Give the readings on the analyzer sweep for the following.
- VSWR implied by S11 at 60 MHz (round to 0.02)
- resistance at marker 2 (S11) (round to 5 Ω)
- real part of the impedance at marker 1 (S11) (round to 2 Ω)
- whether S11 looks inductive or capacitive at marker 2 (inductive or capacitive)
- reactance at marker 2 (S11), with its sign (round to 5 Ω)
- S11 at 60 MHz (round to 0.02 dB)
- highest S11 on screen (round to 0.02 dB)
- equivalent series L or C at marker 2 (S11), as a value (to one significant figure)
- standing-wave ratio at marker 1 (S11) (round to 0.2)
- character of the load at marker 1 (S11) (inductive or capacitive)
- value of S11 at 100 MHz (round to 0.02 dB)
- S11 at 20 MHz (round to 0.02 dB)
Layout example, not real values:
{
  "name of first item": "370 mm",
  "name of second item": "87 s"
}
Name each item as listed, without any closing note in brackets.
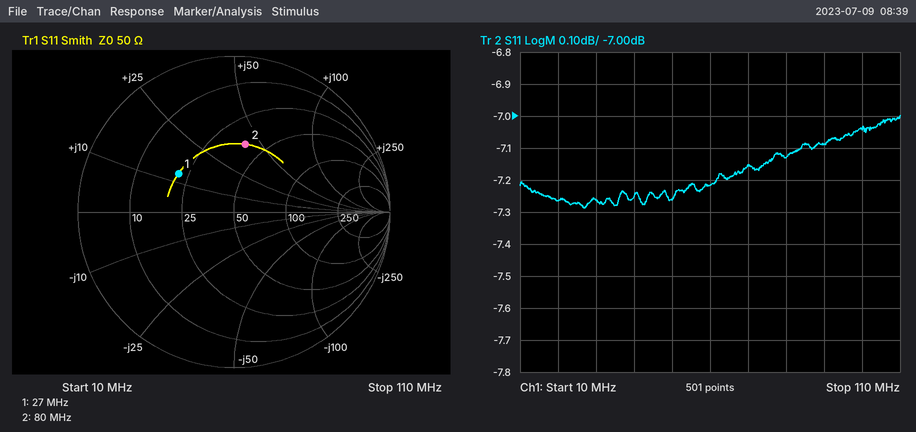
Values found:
{
  "VSWR implied by S11 at 60 MHz": "2.54",
  "resistance at marker 2 (S11)": "40 Ω",
  "real part of the impedance at marker 1 (S11)": "22 Ω",
  "whether S11 looks inductive or capacitive at marker 2": "inductive",
  "reactance at marker 2 (S11), with its sign": "+40 Ω",
  "S11 at 60 MHz": "-7.22 dB",
  "highest S11 on screen": "-7.00 dB",
  "equivalent series L or C at marker 2 (S11), as a value": "80 nH",
  "standing-wave ratio at marker 1 (S11)": "2.6",
  "character of the load at marker 1 (S11)": "inductive",
  "value of S11 at 100 MHz": "-7.04 dB",
  "S11 at 20 MHz": "-7.26 dB"
}
